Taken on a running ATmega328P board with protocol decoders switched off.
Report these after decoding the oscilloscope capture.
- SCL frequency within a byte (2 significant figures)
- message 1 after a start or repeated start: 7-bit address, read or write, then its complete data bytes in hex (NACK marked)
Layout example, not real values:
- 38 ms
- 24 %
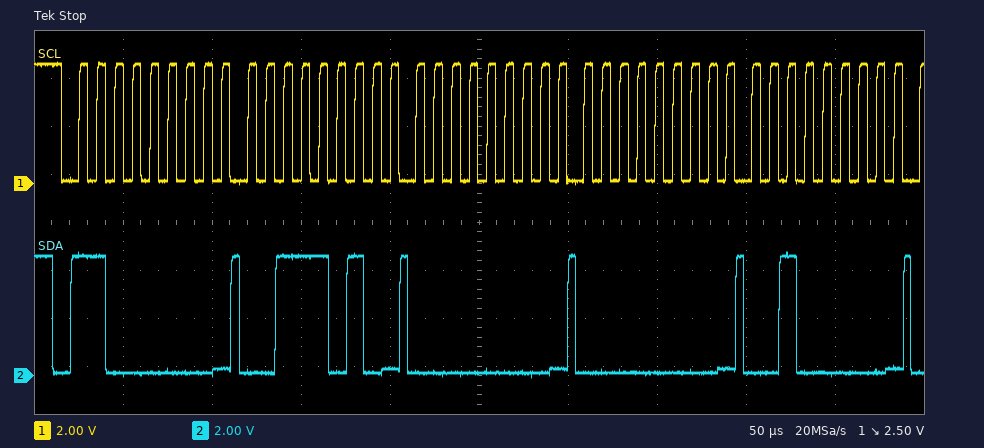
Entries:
- 100 kHz
- 0x60 write: 3A 00 00 20
